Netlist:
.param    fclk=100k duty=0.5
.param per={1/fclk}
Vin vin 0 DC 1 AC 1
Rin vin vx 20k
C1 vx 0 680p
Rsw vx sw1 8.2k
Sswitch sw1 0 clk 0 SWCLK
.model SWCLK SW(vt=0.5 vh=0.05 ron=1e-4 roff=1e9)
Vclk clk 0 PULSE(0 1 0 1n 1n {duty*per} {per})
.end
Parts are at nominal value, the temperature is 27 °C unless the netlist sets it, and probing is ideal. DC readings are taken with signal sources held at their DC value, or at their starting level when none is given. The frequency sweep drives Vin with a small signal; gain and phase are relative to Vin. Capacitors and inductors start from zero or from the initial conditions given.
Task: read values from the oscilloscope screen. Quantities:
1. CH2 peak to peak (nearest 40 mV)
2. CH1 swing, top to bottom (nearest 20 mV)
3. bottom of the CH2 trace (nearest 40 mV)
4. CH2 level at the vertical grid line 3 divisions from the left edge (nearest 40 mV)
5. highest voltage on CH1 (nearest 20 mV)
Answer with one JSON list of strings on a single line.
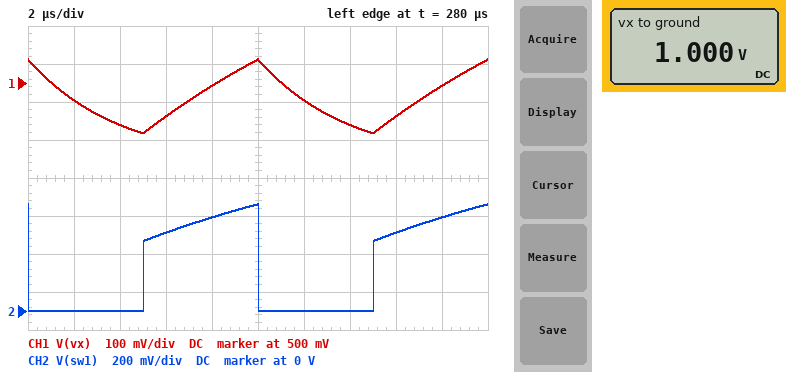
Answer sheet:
["560 mV", "200 mV", "0 V", "400 mV", "560 mV"]
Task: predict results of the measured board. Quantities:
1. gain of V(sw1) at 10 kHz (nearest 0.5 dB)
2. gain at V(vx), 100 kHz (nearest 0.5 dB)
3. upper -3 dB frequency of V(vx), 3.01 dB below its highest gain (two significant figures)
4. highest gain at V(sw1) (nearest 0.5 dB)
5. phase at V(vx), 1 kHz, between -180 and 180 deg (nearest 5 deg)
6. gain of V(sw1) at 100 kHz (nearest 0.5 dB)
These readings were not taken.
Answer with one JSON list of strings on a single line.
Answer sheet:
["-2.5 dB", "-18.5 dB", "12 kHz", "0 dB", "-5 deg", "-18.5 dB"]
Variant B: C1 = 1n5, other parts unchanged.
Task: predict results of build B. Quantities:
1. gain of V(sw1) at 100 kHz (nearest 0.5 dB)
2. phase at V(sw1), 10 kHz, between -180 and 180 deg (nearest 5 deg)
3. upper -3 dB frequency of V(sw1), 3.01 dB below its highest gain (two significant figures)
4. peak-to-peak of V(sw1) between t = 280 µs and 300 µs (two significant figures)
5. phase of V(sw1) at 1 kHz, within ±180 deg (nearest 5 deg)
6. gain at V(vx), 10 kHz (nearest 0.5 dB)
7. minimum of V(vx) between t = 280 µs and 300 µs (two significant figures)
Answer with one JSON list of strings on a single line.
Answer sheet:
["-25.5 dB", "-60 deg", "5.3 kHz", "500 mV", "-10 deg", "-6.5 dB", "410 mV"]
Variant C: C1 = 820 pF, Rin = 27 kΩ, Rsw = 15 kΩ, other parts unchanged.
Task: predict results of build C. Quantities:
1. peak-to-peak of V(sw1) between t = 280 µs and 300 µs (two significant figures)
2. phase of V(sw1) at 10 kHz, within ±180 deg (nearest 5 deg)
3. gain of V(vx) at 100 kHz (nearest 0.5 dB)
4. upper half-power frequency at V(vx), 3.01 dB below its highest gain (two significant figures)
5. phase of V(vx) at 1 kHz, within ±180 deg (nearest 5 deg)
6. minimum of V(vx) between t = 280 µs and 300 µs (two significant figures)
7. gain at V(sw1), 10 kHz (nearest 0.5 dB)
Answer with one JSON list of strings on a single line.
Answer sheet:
["580 mV", "-55 deg", "-23.0 dB", "7.2 kHz", "-10 deg", "480 mV", "-4.5 dB"]
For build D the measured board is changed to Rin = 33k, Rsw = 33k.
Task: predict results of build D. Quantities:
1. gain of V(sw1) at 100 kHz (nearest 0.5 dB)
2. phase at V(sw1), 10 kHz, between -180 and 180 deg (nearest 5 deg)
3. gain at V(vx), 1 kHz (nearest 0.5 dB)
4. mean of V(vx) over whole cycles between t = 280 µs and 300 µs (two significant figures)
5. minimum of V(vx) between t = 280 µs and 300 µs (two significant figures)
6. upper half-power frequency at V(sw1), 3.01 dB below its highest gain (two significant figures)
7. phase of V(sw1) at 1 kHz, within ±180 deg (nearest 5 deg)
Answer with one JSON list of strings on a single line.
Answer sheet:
["-23.0 dB", "-55 deg", "0 dB", "670 mV", "630 mV", "7.1 kHz", "-10 deg"]
